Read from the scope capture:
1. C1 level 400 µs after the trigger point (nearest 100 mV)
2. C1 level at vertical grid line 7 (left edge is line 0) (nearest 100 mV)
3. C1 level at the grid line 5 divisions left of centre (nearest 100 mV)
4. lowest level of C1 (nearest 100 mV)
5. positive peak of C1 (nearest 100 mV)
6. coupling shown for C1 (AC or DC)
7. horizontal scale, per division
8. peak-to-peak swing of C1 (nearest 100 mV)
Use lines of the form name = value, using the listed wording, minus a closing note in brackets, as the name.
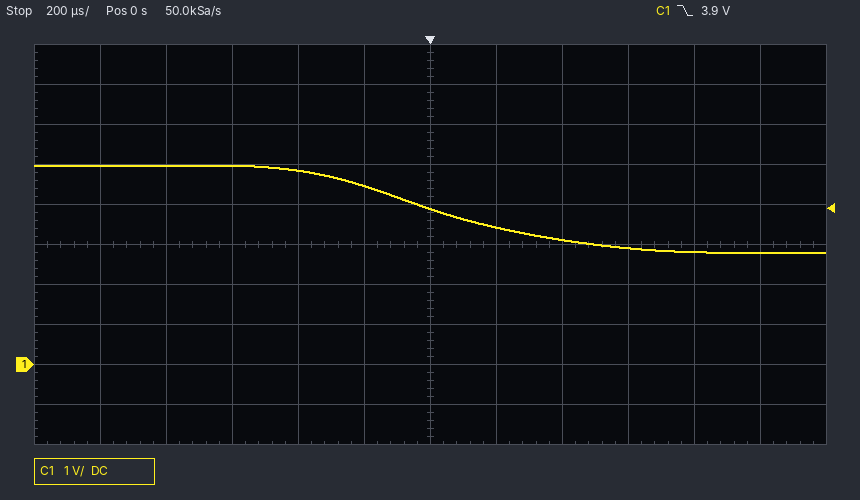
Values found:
C1 level 400 µs after the trigger point = 3.1 V
C1 level at vertical grid line 7 (left edge is line 0) = 3.4 V
C1 level at the grid line 5 divisions left of centre = 5.0 V
lowest level of C1 = 2.8 V
positive peak of C1 = 5.0 V
coupling shown for C1 = DC
horizontal scale, per division = 200 µs
peak-to-peak swing of C1 = 2.2 V
